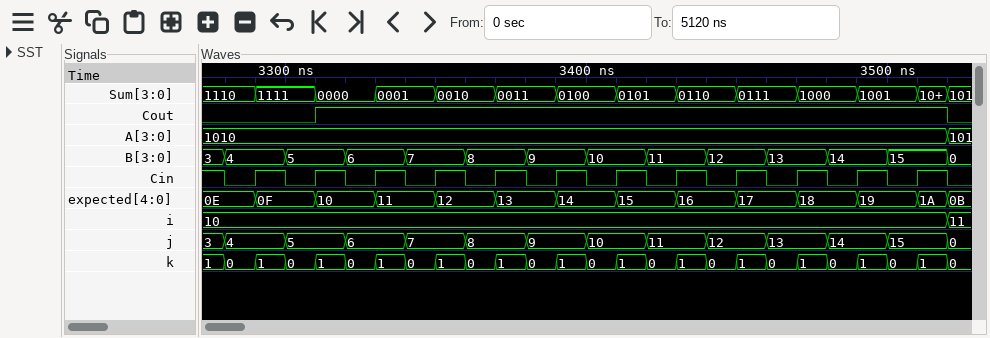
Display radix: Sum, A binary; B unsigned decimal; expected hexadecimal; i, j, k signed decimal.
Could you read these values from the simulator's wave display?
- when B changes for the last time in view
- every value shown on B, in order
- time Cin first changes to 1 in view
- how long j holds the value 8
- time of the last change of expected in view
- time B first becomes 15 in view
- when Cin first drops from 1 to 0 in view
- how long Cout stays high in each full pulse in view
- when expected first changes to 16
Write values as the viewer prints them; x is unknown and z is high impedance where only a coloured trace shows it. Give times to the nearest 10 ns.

3520 ns
3, 4, 5, 6, 7, 8, 9, 10, 11, 12, 13, 14, 15, 0
3290 ns
20 ns
3520 ns
3500 ns
3280 ns
210 ns
3430 ns
